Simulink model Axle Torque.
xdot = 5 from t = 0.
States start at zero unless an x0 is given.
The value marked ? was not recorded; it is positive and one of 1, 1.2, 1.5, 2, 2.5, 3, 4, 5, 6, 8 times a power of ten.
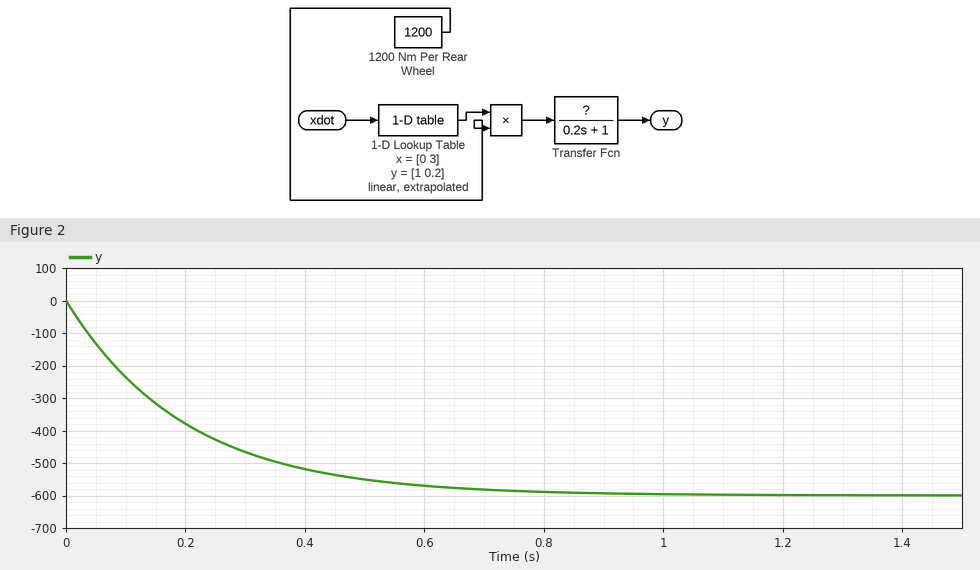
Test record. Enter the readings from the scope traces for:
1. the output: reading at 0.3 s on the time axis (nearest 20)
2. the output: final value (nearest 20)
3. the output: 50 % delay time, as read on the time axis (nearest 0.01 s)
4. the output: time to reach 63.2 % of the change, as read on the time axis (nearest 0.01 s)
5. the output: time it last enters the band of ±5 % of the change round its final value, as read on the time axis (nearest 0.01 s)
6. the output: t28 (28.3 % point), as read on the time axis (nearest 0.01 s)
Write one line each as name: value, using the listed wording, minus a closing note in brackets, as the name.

the output: reading at 0.3 s on the time axis: -460
the output: final value: -600
the output: 50 % delay time, as read on the time axis: 0.14 s
the output: time to reach 63.2 % of the change, as read on the time axis: 0.20 s
the output: time it last enters the band of ±5 % of the change round its final value, as read on the time axis: 0.60 s
the output: t28 (28.3 % point), as read on the time axis: 0.07 s
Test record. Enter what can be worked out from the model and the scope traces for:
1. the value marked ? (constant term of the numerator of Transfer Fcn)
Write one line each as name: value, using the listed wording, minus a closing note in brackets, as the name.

the value marked ?: 1.5
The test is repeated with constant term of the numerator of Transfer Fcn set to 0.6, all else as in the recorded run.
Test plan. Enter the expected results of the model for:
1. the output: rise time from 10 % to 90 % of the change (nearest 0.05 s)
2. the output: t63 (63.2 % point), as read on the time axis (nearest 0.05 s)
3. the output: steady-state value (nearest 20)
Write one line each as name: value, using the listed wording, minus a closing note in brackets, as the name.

the output: rise time from 10 % to 90 % of the change: 0.45 s
the output: t63 (63.2 % point), as read on the time axis: 0.20 s
the output: steady-state value: -240
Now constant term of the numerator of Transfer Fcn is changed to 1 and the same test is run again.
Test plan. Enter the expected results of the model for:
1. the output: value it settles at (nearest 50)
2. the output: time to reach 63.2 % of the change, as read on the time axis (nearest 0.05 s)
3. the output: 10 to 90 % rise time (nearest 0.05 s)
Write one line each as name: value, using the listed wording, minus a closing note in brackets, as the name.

the output: value it settles at: -400
the output: time to reach 63.2 % of the change, as read on the time axis: 0.20 s
the output: 10 to 90 % rise time: 0.45 s
